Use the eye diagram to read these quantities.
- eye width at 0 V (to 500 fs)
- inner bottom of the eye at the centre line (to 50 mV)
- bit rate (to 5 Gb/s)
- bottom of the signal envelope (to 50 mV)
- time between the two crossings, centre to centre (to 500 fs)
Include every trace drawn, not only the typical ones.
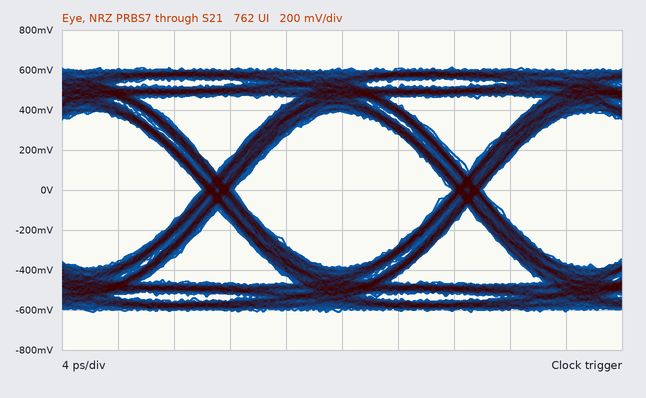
15.5 ps
-400 mV
55 Gb/s
-600 mV
18.0 ps
